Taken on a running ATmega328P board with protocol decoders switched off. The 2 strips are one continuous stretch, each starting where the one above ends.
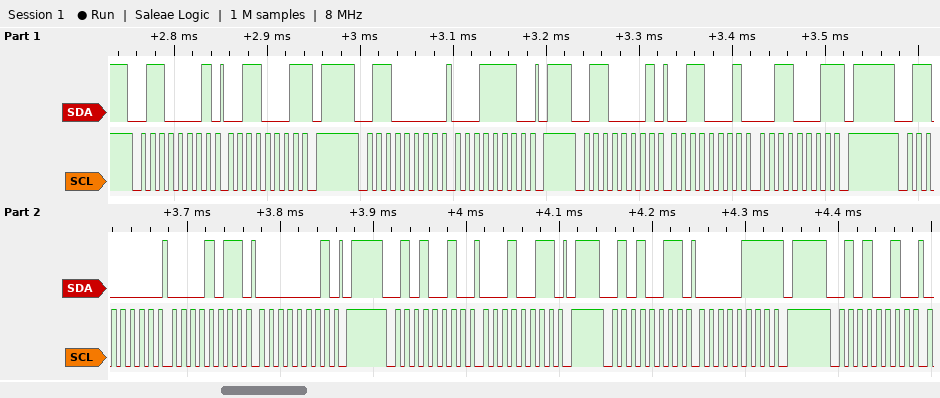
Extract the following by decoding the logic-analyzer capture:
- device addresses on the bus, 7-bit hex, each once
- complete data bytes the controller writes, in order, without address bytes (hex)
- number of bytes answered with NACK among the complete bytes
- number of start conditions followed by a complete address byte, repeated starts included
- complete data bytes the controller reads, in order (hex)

0x30 0x29
1E 0B 01 13
3
7
31 31 31 07
